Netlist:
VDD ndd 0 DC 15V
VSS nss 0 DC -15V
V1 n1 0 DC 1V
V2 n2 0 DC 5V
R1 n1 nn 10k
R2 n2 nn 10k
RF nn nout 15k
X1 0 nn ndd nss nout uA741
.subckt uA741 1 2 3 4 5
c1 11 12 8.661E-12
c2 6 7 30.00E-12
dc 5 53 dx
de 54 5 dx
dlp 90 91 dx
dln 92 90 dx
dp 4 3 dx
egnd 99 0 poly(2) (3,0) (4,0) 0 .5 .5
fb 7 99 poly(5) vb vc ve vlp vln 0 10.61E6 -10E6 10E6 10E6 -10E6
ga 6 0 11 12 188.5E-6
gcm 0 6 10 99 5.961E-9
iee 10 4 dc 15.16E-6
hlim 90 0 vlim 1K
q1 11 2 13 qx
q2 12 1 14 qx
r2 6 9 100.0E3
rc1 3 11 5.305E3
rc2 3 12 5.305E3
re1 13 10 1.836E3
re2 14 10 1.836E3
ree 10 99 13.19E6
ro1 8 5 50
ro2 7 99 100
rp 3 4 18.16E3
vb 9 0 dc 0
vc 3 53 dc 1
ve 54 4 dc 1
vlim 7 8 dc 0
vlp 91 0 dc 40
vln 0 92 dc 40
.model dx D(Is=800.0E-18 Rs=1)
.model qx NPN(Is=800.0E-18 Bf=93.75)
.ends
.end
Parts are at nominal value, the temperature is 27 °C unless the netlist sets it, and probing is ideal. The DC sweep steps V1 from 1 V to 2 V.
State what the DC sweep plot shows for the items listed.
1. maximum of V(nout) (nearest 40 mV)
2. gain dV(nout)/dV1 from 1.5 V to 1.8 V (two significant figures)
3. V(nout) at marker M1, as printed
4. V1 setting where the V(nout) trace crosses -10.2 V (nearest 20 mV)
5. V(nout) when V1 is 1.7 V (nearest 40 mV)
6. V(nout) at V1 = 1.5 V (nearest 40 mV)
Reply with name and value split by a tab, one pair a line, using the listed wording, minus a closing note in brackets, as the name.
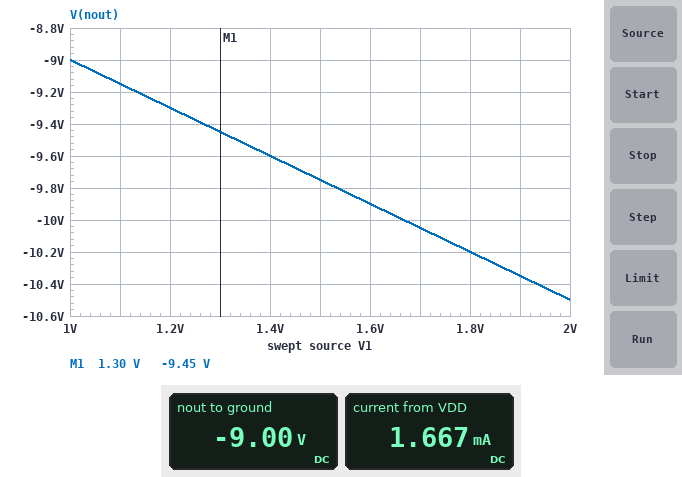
maximum of V(nout)	-9.00 V
gain dV(nout)/dV1 from 1.5 V to 1.8 V	-1.5 V/V
V(nout) at marker M1, as printed	-9.45 V
V1 setting where the V(nout) trace crosses -10.2 V	1.80 V
V(nout) when V1 is 1.7 V	-10.04 V
V(nout) at V1 = 1.5 V	-9.76 V
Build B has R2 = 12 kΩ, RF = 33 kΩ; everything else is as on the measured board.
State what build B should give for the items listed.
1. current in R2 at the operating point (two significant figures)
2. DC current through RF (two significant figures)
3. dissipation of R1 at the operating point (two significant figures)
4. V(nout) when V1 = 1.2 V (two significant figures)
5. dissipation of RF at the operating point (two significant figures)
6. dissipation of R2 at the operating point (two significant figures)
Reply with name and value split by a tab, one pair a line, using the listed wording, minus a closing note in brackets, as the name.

current in R2 at the operating point	390 µA
DC current through RF	450 µA
dissipation of R1 at the operating point	43 µW
V(nout) when V1 = 1.2 V	-15 V
dissipation of RF at the operating point	6.8 mW
dissipation of R2 at the operating point	1.8 mW
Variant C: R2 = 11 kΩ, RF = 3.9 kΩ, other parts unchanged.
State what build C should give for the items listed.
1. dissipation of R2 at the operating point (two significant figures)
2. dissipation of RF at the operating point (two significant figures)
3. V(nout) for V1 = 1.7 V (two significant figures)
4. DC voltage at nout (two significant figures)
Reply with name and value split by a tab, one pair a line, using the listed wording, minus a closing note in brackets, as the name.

dissipation of R2 at the operating point	2.3 mW
dissipation of RF at the operating point	1.2 mW
V(nout) for V1 = 1.7 V	-2.4 V
DC voltage at nout	-2.2 V
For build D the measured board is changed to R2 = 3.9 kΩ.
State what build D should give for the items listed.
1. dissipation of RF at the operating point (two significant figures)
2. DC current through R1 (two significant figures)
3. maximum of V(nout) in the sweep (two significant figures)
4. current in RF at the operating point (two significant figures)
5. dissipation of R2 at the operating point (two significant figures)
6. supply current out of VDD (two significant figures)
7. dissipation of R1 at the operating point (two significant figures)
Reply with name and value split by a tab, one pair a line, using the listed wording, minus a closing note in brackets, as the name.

dissipation of RF at the operating point	16 mW
DC current through R1	3.6 µA
maximum of V(nout) in the sweep	-15 V
current in RF at the operating point	1.0 mA
dissipation of R2 at the operating point	4.2 mW
supply current out of VDD	1.7 mA
dissipation of R1 at the operating point	130 nW
